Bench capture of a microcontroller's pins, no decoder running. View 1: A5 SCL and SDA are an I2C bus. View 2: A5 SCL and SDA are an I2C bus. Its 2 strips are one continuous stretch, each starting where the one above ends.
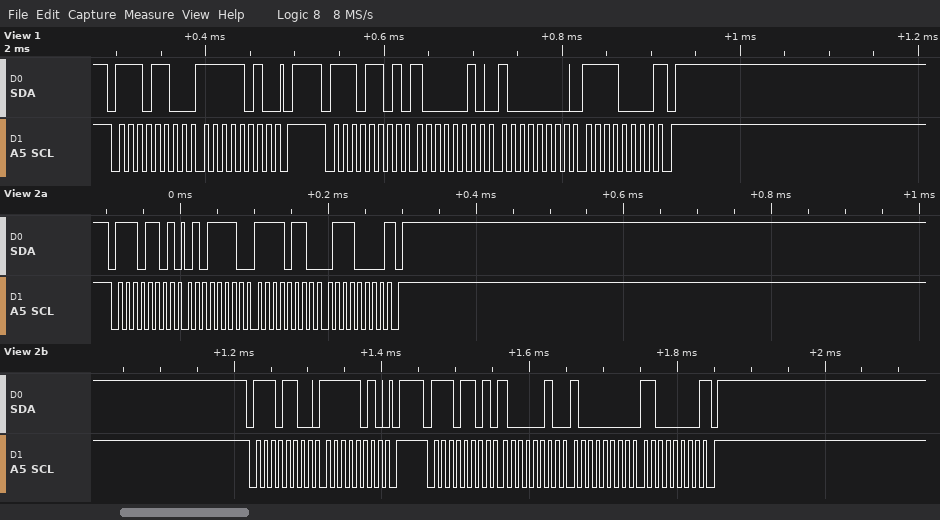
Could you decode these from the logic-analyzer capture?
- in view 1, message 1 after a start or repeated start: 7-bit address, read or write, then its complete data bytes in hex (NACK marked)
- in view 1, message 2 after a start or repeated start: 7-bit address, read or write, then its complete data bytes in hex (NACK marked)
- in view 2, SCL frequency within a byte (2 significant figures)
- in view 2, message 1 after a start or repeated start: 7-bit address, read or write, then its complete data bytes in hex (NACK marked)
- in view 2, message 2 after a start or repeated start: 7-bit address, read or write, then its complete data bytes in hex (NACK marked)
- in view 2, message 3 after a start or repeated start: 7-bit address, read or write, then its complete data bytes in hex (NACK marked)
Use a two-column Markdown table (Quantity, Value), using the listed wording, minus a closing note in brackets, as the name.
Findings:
| Quantity | Value |
|---|---|
| in view 1, message 1 after a start or repeated start: 7-bit address, read or write, then its complete data bytes in hex | 0x76 write: FA |
| in view 1, message 2 after a start or repeated start: 7-bit address, read or write, then its complete data bytes in hex | 0x76 read: 82 80 F0 NACK |
| in view 2, SCL frequency within a byte | 100 kHz |
| in view 2, message 1 after a start or repeated start: 7-bit address, read or write, then its complete data bytes in hex | 0x76 read: 5E F6 70 NACK |
| in view 2, message 2 after a start or repeated start: 7-bit address, read or write, then its complete data bytes in hex | 0x76 write: FA |
| in view 2, message 3 after a start or repeated start: 7-bit address, read or write, then its complete data bytes in hex | 0x76 read: 82 80 C0 NACK |
